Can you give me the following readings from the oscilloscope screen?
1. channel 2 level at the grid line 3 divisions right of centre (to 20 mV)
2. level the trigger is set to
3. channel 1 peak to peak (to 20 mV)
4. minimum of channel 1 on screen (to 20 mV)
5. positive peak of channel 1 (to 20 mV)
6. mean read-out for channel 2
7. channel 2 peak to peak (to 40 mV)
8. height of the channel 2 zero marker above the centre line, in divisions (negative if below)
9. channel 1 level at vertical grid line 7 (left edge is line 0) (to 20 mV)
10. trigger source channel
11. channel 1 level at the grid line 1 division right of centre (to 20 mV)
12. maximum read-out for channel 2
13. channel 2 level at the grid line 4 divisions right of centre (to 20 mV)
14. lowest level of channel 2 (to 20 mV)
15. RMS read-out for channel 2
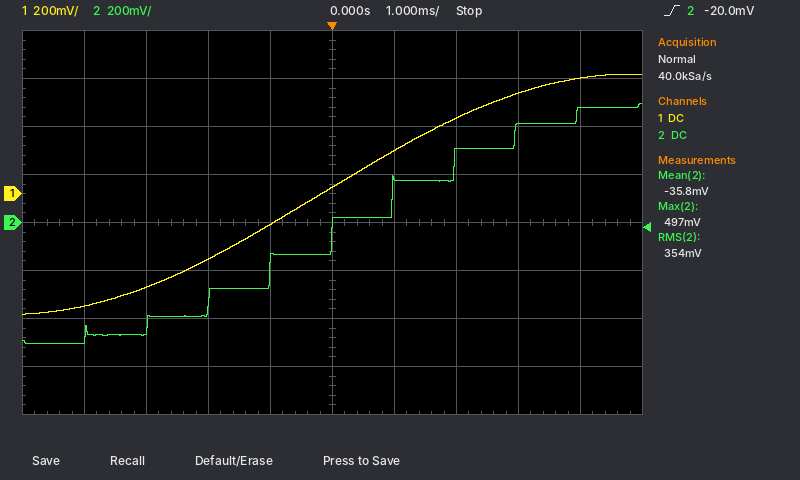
400 mV
-20.0 mV
1.00 V
-500 mV
500 mV
-35.8 mV
1.00 V
0.0 div
320 mV
channel 2
180 mV
497 mV
480 mV
-500 mV
354 mV
